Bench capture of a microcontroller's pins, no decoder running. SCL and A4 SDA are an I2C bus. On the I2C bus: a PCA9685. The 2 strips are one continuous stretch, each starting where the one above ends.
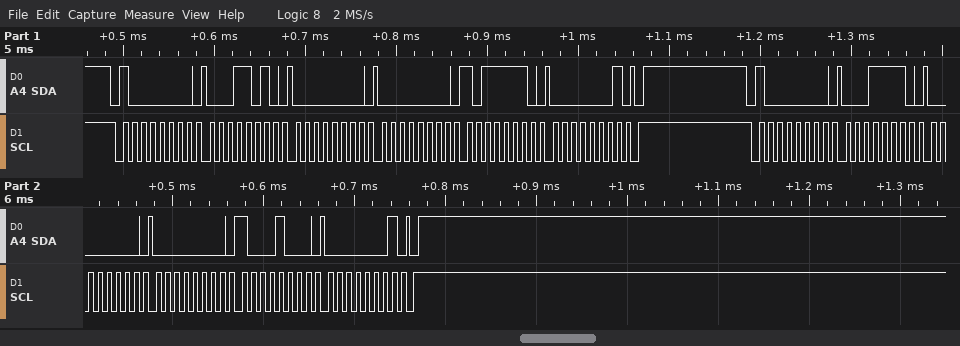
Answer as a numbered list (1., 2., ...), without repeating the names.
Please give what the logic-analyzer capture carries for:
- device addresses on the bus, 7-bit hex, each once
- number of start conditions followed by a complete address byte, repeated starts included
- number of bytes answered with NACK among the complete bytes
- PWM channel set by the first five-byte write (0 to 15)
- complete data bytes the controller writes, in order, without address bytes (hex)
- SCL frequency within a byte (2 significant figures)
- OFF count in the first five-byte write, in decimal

1. 0x40
2. 2
3. 0
4. 5
5. 1A 00 00 BE 01 1E 00 00 88 01
6. 100 kHz
7. 446
